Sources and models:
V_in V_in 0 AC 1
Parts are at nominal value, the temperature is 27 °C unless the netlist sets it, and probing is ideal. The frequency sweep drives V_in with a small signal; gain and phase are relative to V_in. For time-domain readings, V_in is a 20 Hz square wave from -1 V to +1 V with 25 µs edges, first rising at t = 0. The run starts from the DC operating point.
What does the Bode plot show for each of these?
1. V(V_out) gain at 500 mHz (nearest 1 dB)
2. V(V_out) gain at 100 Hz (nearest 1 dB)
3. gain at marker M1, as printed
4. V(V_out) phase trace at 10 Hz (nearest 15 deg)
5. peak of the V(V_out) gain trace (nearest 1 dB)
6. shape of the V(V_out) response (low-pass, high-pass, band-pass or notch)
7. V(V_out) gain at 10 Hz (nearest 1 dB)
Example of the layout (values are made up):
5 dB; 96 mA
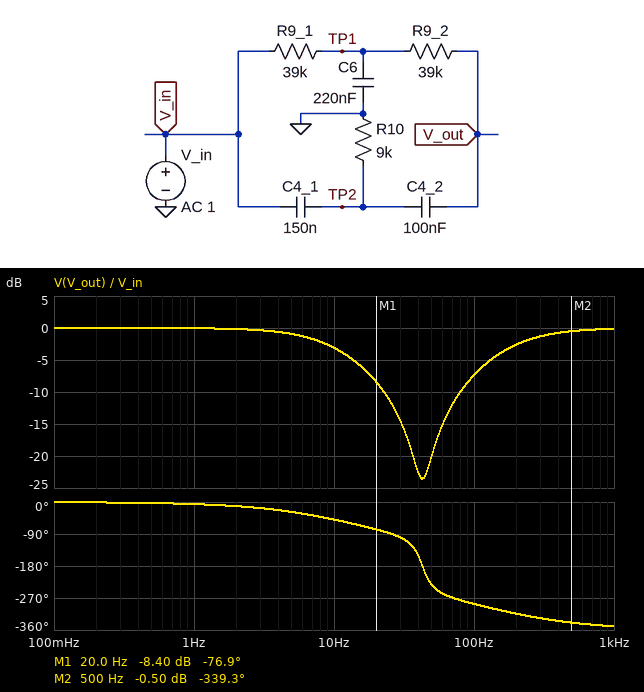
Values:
0 dB; -7 dB; -8.40 dB; -45 deg; 0 dB; notch; -3 dB
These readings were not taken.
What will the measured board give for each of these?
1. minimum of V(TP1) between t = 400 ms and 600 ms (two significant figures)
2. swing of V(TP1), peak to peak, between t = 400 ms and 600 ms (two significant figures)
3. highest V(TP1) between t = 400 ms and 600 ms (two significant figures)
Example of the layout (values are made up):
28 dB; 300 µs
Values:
-740 mV; 1.5 V; 740 mV
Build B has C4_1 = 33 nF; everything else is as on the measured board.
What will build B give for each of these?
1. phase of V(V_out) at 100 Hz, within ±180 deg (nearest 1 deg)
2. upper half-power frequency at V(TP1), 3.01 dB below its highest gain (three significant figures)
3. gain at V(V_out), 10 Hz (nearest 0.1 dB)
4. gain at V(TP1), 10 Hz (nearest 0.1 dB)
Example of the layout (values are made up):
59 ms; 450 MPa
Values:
119 deg; 11.7 Hz; -2.8 dB; -2.4 dB
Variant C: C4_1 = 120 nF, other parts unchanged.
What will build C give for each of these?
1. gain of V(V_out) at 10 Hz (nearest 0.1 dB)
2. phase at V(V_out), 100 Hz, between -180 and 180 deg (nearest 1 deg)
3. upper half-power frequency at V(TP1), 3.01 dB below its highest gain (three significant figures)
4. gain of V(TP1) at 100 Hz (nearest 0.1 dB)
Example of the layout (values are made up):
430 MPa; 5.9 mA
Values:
-3.0 dB; 80 deg; 11.4 Hz; -14.2 dB
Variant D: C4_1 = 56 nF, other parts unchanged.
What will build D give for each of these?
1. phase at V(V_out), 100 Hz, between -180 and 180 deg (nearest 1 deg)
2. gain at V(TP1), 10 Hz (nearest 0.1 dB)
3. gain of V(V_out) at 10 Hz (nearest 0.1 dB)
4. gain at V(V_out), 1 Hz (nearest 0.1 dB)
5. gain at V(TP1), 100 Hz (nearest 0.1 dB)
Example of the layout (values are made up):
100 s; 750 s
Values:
101 deg; -2.4 dB; -2.9 dB; 0 dB; -15.4 dB
